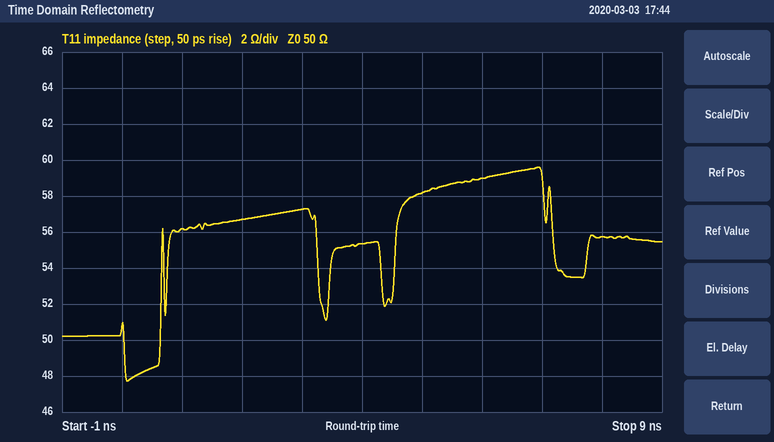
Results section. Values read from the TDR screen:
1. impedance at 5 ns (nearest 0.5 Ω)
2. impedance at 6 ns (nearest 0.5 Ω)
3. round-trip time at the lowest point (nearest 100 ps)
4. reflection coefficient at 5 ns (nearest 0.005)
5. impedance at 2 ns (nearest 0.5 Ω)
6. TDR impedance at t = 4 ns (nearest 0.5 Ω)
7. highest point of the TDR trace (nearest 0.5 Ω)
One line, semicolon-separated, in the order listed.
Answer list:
58.0 Ω; 59.0 Ω; 100 ps; +0.075; 56.5 Ω; 55.5 Ω; 59.5 Ω
